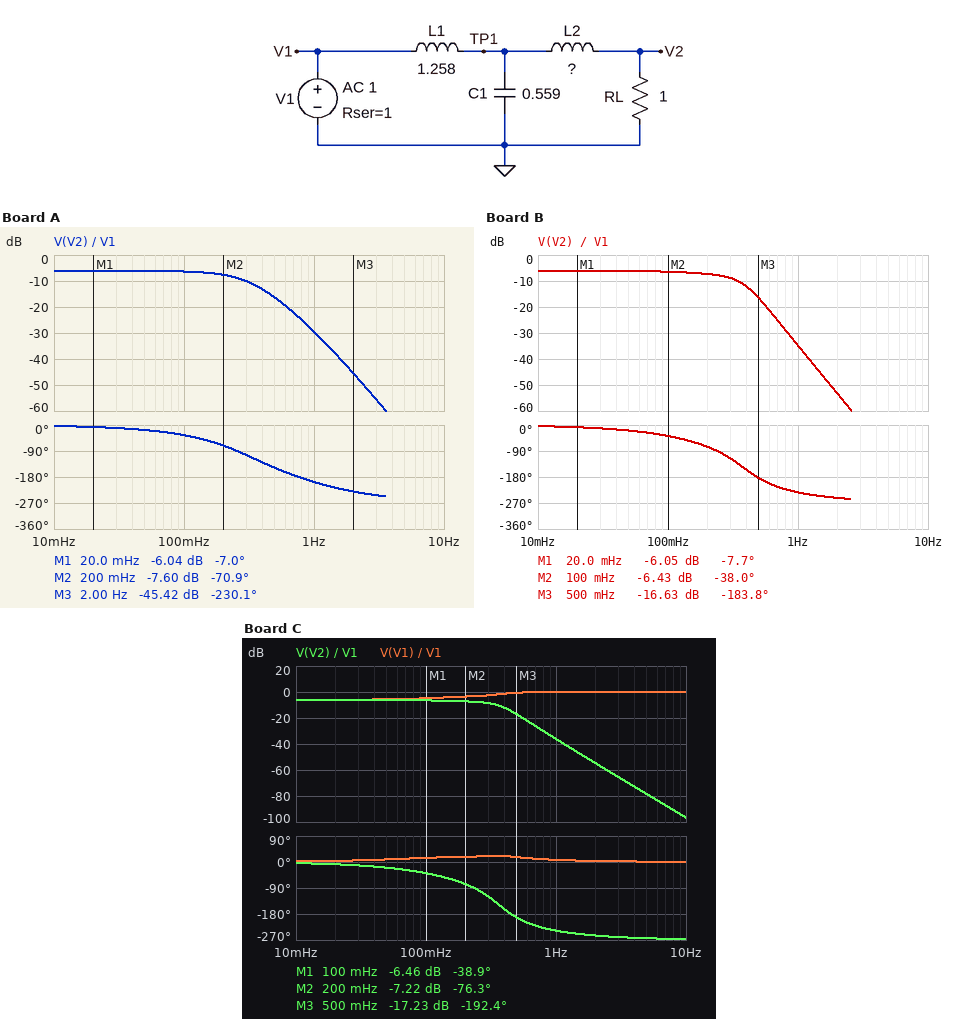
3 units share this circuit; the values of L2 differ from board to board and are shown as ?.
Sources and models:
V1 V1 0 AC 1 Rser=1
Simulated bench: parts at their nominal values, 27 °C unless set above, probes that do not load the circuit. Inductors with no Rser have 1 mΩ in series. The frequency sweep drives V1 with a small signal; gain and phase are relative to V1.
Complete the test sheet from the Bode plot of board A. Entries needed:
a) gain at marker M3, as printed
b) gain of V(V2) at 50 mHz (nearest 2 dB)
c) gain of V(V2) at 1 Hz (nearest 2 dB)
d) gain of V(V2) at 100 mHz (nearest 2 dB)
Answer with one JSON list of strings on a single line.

["-45.42 dB", "-6 dB", "-30 dB", "-6 dB"]
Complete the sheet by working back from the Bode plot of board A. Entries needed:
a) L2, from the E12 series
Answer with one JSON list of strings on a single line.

["120 mH"]
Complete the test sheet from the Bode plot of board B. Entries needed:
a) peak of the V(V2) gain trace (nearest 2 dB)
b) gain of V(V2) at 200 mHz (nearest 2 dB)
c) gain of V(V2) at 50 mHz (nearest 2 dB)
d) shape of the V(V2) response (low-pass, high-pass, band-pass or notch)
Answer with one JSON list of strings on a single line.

["-6 dB", "-8 dB", "-6 dB", "low-pass"]
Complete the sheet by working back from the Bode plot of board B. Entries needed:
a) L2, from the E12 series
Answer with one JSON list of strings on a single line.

["330 mH"]
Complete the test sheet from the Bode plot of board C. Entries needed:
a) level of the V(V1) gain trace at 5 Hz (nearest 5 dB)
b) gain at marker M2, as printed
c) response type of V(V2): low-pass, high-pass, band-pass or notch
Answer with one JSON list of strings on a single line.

["0 dB", "-7.22 dB", "low-pass"]
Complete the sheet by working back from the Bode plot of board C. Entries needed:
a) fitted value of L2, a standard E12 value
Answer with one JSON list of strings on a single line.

["390 mH"]
